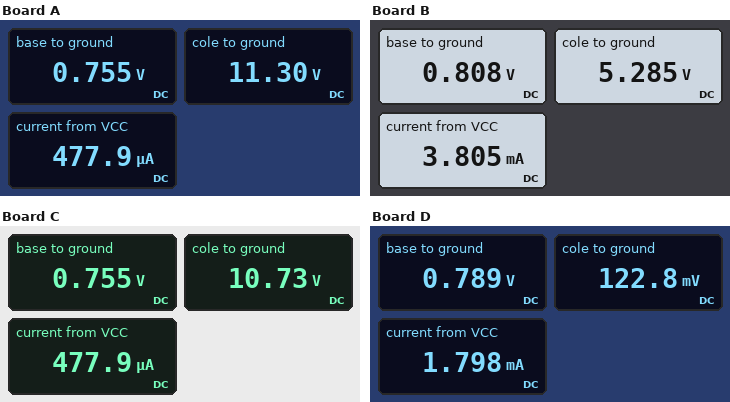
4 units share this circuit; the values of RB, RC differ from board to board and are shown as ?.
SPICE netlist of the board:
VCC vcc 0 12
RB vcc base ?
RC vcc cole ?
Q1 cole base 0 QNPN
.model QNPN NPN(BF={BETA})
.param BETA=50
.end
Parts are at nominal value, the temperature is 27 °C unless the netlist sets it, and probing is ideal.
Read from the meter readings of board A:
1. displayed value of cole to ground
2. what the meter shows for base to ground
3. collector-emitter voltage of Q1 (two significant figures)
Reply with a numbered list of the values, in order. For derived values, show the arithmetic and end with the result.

1. 11.30 V
2. 0.755 V
3. 11.3 V = 11 V
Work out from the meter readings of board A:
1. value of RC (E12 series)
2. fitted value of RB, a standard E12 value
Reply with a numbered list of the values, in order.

1. 1.5 kΩ
2. 1.2 MΩ
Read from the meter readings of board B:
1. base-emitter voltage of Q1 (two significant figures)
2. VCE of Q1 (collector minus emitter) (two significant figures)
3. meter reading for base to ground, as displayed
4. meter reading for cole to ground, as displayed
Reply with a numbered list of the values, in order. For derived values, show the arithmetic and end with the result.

1. 808 mV = 810 mV
2. 5.285 V = 5.3 V
3. 0.808 V
4. 5.285 V
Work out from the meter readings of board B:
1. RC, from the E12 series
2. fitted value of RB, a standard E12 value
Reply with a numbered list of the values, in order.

1. 1.8 kΩ
2. 150 kΩ
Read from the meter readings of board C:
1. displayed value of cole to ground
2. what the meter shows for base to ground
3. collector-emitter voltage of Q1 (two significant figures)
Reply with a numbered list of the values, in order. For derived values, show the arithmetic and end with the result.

1. 10.73 V
2. 0.755 V
3. 10.73 V = 11 V
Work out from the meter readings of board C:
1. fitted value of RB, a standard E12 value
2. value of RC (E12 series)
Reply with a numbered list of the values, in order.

1. 1.2 MΩ
2. 2.7 kΩ
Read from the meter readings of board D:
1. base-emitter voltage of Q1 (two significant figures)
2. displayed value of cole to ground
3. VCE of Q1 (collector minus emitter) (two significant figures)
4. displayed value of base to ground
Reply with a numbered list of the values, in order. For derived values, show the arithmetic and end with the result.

1. 789 mV = 790 mV
2. 122.8 mV
3. 122.8 mV = 120 mV
4. 0.789 V
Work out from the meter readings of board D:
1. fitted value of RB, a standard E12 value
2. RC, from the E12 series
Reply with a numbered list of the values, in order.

1. 220 kΩ
2. 6.8 kΩ
